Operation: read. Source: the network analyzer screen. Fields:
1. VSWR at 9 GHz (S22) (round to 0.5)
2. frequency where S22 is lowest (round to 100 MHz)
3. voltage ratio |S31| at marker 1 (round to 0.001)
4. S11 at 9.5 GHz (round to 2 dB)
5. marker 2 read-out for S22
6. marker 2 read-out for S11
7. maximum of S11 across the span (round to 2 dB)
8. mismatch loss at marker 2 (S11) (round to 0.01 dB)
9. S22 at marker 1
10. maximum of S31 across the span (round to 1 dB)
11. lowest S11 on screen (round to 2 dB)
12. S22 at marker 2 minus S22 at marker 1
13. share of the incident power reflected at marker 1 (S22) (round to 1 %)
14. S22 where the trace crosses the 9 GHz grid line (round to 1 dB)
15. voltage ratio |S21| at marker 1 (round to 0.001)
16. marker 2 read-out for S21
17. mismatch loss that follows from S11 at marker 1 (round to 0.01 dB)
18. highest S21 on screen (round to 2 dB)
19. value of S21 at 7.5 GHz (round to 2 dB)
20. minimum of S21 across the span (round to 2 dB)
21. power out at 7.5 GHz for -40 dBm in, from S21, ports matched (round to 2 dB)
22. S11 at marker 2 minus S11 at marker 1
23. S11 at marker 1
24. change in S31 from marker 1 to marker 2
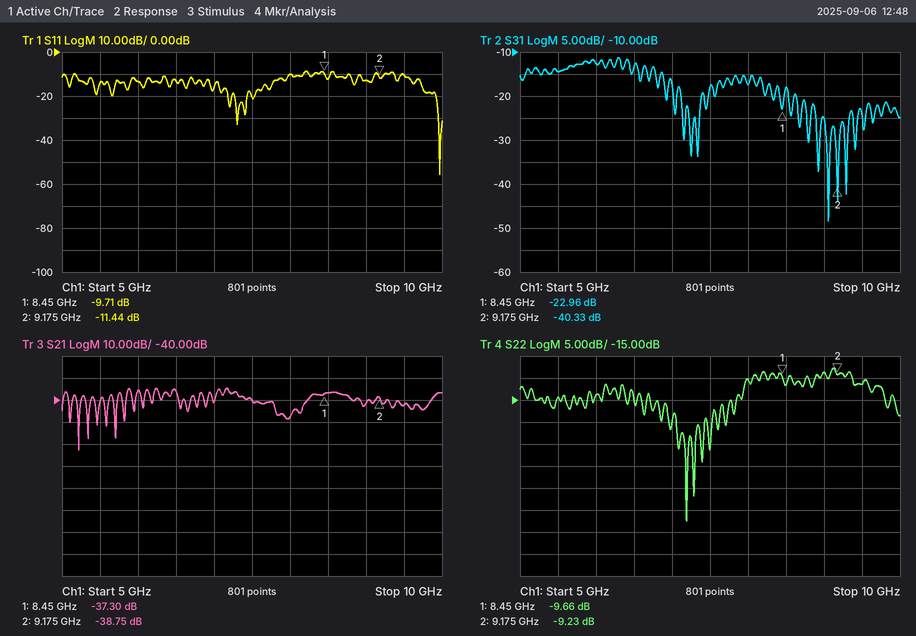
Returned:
2.0
7.2 GHz
0.071
-10 dB
-9.23 dB
-11.44 dB
-8 dB
0.32 dB
-9.66 dB
-11 dB
-56 dB
0.43 dB
11 %
-9 dB
0.014
-38.75 dB
0.49 dB
-34 dB
-40 dB
-62 dB
-80 dBm
-1.73 dB
-9.71 dB
-17.37 dB
